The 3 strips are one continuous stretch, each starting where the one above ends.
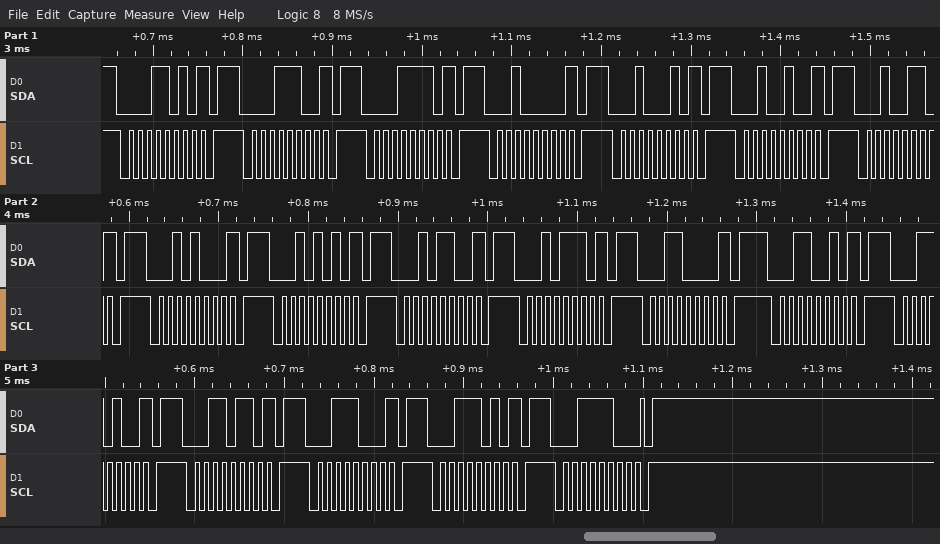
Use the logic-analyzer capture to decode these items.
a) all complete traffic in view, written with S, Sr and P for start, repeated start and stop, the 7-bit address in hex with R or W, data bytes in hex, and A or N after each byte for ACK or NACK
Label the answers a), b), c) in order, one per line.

a) S 0DW N P S 0EW N P S 0FW N P S 10W N P S 11W N P S 12W N P S 13W N P S 14W N P S 15W N P S 16W N P S 17W N P S 18W N P S 19W N P S 1AW N P S 1BW N P S 1CW N P S 1DW N P S 1EW A P
